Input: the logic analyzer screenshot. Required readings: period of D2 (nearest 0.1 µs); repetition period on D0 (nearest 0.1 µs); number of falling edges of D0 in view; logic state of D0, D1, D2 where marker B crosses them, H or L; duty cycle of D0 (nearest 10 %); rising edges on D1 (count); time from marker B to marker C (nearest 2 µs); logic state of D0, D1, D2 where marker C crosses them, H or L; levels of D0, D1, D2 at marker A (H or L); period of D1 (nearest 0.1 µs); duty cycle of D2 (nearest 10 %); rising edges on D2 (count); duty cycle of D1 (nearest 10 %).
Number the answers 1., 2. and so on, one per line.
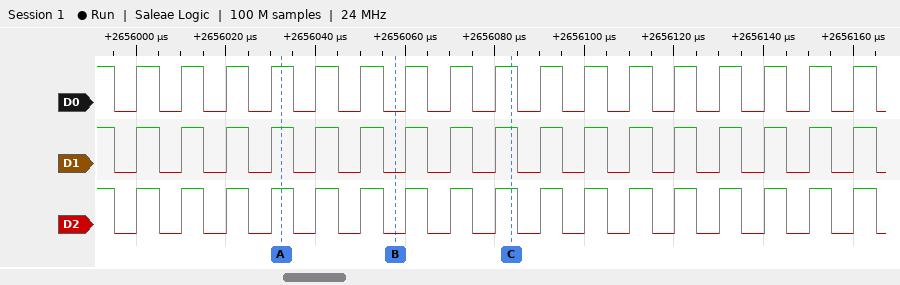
1. 10 µs
2. 10 µs
3. 18
4. D0=L, D1=L, D2=L
5. 50 %
6. 17
7. 26 µs
8. D0=H, D1=H, D2=H
9. D0=H, D1=H, D2=H
10. 10 µs
11. 50 %
12. 17
13. 50 %
